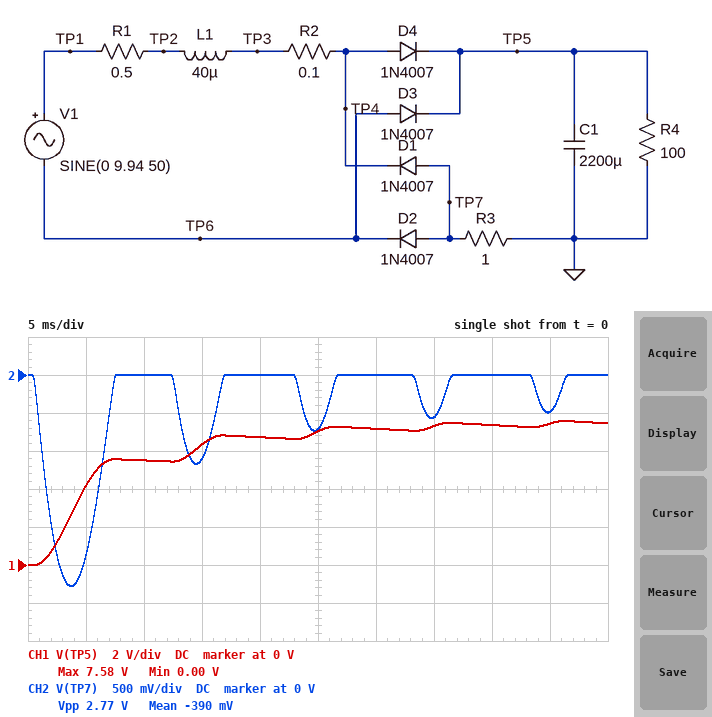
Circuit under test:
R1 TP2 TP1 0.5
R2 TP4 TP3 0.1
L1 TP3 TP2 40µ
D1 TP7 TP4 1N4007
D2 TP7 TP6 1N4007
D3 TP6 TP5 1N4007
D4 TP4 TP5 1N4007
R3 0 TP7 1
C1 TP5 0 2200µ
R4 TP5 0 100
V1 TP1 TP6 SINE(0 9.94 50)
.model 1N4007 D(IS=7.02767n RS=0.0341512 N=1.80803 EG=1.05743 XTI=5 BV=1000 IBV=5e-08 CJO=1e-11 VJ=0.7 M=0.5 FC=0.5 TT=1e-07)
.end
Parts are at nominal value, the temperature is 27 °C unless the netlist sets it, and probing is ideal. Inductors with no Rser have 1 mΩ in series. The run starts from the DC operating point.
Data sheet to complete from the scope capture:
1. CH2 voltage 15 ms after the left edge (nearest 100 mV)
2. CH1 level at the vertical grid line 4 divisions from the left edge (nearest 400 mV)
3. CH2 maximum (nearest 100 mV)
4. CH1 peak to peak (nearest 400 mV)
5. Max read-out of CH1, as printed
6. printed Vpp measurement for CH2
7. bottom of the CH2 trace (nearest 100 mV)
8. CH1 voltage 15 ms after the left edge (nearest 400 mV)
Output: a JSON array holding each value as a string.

["-1.1 V", "6.8 V", "0 V", "7.6 V", "7.58 V", "2.77 V", "-2.8 V", "6.4 V"]
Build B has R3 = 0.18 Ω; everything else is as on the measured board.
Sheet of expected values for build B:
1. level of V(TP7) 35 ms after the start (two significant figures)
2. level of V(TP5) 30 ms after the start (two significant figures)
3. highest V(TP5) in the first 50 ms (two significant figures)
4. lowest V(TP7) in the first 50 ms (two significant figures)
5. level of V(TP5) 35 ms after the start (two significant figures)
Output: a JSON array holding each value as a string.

["-100 mV", "7.7 V", "7.9 V", "-700 mV", "7.8 V"]
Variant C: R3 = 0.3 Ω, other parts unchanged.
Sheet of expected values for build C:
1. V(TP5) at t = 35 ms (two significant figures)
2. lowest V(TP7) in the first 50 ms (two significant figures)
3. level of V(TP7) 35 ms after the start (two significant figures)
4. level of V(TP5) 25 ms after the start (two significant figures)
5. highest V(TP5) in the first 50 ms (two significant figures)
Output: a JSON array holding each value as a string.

["7.7 V", "-1.1 V", "-170 mV", "7.6 V", "7.9 V"]
